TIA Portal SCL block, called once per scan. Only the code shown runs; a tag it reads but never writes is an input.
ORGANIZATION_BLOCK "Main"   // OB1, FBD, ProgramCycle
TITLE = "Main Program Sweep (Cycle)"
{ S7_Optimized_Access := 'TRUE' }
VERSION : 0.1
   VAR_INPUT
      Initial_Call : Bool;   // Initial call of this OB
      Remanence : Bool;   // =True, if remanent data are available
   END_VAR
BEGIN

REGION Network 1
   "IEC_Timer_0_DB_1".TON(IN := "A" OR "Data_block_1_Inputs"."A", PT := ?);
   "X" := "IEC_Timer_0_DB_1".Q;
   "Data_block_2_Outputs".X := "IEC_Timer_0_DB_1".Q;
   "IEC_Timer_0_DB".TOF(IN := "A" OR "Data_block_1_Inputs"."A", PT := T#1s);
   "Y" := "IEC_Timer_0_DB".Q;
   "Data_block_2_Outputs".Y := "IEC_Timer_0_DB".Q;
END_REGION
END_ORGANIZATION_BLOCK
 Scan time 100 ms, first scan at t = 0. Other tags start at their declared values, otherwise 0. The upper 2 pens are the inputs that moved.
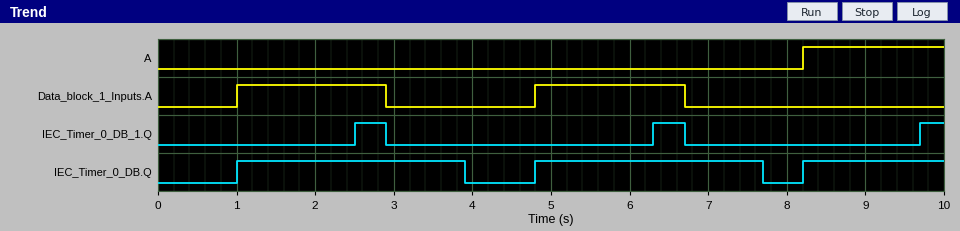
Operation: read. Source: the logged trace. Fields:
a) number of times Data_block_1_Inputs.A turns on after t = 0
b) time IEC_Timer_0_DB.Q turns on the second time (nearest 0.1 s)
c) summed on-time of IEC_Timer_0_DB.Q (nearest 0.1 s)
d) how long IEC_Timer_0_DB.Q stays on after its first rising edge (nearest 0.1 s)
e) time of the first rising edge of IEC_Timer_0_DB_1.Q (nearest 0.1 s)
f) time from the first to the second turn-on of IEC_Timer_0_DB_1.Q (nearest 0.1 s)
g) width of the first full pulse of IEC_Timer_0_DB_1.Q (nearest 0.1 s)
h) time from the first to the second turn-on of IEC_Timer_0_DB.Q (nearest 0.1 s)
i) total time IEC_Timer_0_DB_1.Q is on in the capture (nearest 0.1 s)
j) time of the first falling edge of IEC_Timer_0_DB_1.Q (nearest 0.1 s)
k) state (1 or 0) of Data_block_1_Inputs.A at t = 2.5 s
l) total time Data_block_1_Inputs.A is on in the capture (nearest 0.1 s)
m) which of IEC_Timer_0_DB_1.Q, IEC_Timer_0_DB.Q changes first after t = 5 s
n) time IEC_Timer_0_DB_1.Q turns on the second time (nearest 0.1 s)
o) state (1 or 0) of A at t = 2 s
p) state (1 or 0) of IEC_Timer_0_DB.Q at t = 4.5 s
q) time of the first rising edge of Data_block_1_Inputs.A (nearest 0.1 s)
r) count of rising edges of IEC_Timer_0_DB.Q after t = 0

2
4.8 s
7.6 s
2.9 s
2.5 s
3.8 s
0.4 s
3.8 s
1.1 s
2.9 s
1
3.8 s
IEC_Timer_0_DB_1.Q
6.3 s
0
0
1.0 s
3
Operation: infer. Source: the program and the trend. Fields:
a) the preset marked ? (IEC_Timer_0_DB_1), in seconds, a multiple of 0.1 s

1.5 s
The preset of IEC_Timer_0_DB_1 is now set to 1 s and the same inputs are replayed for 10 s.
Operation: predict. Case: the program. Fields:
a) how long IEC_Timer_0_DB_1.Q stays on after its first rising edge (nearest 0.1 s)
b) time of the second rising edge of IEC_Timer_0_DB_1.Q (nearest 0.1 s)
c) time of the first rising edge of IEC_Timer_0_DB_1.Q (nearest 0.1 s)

0.9 s
5.8 s
2.0 s
